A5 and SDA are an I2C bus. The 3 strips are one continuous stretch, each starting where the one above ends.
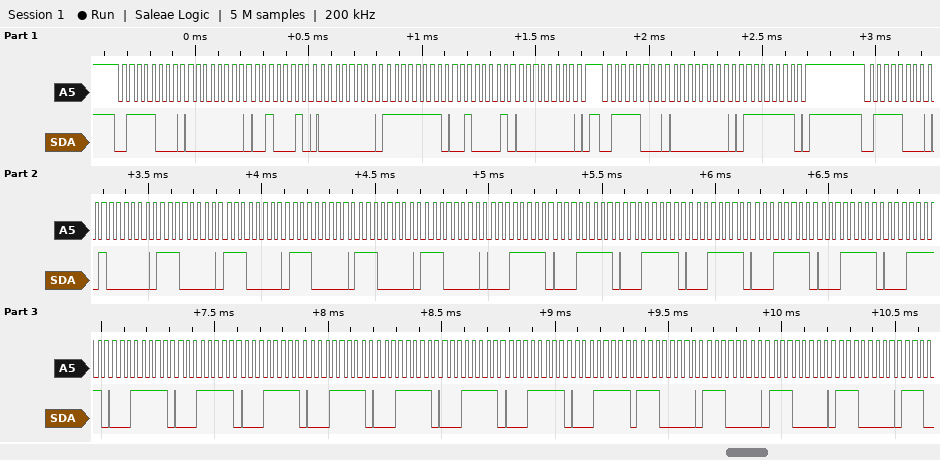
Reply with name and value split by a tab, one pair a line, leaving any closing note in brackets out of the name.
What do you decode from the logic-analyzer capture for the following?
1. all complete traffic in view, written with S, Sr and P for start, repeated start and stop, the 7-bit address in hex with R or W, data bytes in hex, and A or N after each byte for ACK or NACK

all complete traffic in view, written with S, Sr and P for start, repeated start and stop, the 7-bit address in hex with R or W, data bytes in hex, and A or N after each byte for ACK or NACK	S 3CW A 00 A 22 A 00 A FF A 21 A 00 A P S 3CW A 00 A 7F A P S 3CW A 40 A E0 A E0 A E0 A E0 A E0 A 1F A 1F A 1F A 1F A 1F A 1F A 1F A 1F A 1F A 1F A 1F A 1F A 1F A 1F A 1F A E0 A E0 A E0 A E0 A
